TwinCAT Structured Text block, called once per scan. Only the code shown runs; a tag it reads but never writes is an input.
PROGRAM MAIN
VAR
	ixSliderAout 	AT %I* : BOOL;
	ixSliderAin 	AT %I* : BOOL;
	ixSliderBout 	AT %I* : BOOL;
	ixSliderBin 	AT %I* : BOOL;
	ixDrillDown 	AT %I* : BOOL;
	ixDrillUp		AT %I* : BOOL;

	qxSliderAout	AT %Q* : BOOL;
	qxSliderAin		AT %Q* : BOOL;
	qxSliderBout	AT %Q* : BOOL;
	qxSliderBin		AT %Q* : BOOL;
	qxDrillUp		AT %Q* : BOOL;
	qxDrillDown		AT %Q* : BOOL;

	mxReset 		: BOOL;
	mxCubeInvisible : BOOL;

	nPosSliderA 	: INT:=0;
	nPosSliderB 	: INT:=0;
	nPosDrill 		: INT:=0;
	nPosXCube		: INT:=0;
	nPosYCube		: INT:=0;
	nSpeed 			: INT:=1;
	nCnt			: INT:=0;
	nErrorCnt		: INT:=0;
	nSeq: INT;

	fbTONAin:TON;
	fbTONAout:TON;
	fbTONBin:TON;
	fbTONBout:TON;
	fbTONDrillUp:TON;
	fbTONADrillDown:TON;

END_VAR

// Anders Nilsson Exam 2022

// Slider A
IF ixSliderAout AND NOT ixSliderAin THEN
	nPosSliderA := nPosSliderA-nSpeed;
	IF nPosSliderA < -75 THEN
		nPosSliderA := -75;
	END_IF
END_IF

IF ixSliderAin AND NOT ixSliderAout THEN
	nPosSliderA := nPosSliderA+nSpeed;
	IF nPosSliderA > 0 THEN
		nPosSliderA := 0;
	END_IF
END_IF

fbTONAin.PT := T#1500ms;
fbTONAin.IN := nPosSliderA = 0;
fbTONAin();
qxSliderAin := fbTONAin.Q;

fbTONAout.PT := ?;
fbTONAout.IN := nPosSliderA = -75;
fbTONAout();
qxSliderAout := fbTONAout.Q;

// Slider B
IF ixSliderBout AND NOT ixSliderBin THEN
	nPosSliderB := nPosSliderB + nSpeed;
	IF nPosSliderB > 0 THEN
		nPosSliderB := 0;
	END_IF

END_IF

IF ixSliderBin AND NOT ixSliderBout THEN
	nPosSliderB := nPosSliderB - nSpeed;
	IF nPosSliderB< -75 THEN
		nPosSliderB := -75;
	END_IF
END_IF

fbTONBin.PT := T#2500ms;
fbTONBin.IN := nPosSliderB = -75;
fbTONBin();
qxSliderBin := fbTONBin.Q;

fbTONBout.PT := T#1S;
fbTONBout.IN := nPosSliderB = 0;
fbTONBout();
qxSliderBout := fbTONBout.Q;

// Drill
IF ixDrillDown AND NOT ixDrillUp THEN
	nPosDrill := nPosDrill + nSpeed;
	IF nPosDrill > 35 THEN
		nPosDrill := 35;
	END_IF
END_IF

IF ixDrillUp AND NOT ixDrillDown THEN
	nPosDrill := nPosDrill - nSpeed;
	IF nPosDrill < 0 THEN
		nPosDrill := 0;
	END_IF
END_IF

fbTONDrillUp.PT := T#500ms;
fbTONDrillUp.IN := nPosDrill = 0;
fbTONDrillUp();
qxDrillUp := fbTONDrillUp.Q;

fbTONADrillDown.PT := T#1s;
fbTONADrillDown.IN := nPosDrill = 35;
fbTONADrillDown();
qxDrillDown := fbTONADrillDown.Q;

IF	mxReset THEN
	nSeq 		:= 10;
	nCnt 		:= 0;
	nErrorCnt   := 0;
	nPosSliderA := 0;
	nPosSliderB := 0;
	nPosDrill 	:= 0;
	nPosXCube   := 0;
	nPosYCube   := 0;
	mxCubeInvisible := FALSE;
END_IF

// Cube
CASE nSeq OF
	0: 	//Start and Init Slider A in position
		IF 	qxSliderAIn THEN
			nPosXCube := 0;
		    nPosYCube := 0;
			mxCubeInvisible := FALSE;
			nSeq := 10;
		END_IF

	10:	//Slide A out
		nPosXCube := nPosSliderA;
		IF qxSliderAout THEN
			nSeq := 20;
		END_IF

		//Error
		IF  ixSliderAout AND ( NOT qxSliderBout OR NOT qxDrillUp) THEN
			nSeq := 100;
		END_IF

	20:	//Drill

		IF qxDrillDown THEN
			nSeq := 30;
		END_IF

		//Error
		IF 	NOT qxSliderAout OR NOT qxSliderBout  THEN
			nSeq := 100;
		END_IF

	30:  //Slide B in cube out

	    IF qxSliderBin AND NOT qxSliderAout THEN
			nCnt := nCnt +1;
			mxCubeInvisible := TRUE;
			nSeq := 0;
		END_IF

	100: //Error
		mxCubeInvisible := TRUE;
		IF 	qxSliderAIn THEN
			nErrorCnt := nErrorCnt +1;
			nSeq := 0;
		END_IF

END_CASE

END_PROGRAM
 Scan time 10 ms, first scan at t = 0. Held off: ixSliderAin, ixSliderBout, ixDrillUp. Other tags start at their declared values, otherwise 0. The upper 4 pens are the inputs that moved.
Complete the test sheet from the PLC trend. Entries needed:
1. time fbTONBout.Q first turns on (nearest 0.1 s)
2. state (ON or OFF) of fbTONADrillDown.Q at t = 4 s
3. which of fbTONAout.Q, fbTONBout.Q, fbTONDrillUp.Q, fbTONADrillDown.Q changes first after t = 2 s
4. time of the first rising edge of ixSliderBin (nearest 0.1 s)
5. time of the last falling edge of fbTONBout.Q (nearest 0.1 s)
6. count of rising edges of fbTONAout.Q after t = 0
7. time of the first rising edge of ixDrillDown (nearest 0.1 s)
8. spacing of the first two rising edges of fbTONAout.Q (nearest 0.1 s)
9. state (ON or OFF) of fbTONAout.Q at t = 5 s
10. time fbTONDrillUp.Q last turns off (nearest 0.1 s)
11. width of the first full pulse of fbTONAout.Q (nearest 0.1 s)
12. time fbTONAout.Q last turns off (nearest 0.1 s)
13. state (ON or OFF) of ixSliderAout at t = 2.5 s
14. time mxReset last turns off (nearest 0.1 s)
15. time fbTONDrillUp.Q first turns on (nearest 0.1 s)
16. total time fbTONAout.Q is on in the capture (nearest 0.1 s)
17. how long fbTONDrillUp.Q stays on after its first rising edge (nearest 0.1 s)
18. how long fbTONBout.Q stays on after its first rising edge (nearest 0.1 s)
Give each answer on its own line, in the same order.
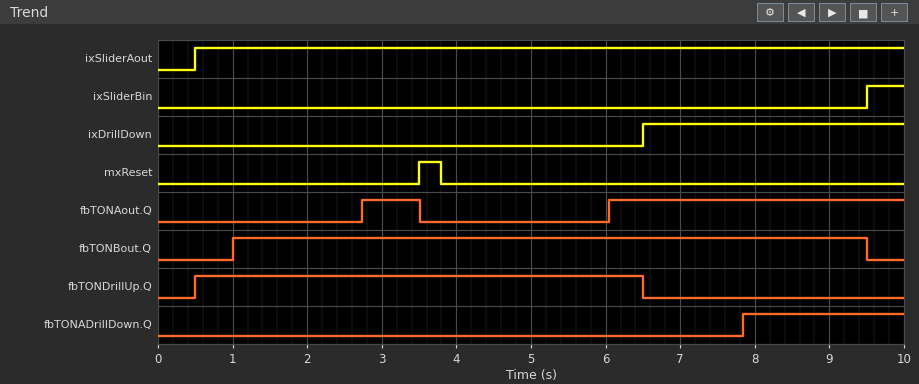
1.0 s
OFF
fbTONAout.Q
9.5 s
9.5 s
2
6.5 s
3.3 s
OFF
6.5 s
0.8 s
3.5 s
ON
3.8 s
0.5 s
4.7 s
6.0 s
8.5 s
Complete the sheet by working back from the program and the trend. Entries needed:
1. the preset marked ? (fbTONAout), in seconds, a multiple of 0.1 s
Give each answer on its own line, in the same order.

1.5 s
